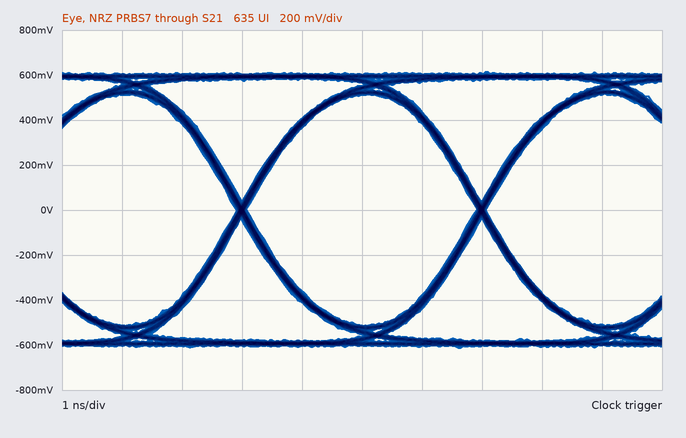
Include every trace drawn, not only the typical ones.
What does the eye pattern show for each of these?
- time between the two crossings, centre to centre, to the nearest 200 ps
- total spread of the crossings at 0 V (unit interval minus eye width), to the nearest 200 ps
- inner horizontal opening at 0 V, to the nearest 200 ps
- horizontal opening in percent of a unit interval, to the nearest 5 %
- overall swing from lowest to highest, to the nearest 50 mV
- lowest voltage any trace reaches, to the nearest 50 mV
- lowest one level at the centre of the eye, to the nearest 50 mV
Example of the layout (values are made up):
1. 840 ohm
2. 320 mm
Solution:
1. 4.0 ns
2. 200 ps
3. 3.8 ns
4. 95 %
5. 1.25 V
6. -600 mV
7. 500 mV
